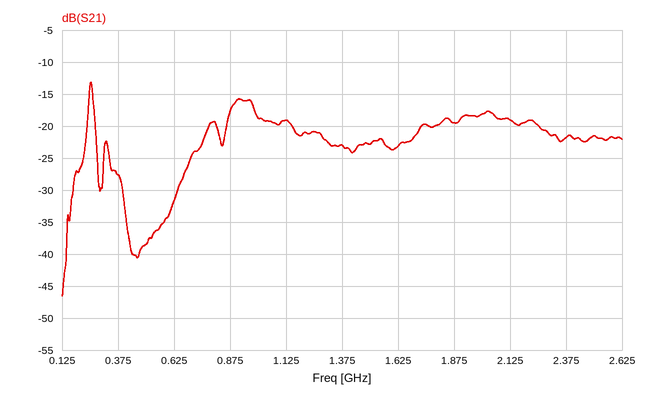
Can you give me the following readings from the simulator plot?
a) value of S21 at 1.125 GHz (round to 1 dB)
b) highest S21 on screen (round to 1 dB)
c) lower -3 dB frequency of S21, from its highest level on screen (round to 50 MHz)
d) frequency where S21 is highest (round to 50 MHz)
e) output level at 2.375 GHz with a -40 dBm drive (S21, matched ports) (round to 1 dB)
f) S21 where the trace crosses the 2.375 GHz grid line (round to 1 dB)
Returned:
-19 dB
-13 dB
250 MHz
250 MHz
-62 dBm
-22 dB
